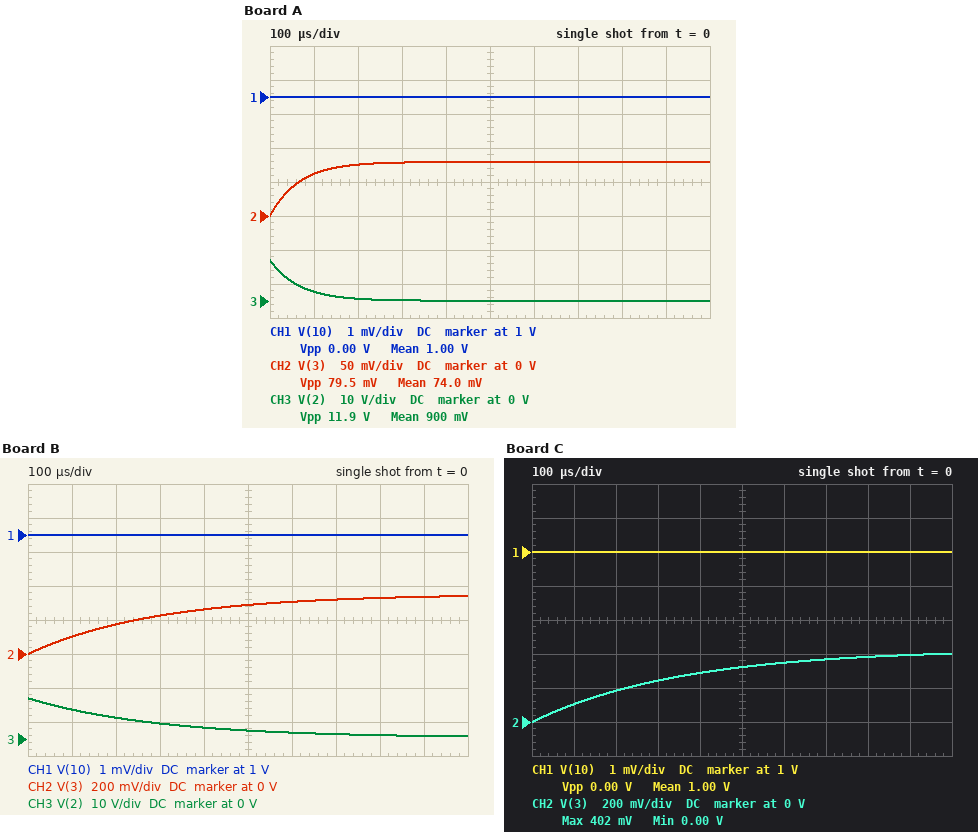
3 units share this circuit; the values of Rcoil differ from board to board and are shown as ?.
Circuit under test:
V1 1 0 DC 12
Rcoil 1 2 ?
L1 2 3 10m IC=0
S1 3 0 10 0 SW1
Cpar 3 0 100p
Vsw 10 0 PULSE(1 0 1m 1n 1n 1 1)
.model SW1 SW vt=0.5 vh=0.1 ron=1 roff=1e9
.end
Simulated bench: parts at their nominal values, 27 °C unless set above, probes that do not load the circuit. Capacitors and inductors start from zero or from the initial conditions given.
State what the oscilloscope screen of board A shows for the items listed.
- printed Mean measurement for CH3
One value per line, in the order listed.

900 mV
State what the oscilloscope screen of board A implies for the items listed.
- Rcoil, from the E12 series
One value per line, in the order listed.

150 Ω
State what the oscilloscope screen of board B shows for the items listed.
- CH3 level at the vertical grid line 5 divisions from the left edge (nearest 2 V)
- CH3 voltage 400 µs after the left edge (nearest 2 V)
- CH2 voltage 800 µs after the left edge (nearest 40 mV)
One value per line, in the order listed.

2 V
4 V
320 mV
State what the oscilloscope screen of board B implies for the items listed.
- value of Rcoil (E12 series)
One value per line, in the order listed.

33 Ω
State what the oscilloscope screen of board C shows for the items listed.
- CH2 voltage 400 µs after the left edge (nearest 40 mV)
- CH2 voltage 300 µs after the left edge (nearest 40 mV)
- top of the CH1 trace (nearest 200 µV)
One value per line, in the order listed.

280 mV
240 mV
1.0000 V
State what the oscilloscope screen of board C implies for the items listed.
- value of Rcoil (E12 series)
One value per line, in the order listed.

27 Ω
